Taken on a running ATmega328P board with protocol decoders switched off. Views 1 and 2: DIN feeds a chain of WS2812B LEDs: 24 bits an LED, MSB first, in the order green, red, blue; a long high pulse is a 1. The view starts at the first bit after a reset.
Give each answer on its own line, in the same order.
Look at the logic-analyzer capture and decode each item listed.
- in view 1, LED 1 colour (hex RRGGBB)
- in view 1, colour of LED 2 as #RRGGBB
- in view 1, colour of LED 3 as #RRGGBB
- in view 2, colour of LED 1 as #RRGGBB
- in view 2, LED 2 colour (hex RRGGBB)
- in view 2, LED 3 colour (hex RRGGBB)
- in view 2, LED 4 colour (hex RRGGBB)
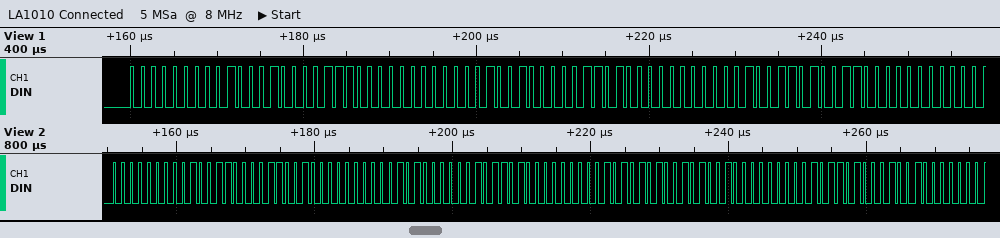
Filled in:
#440038
#480034
#4D0030
#4C0032
#50002D
#550029
#5A0024
